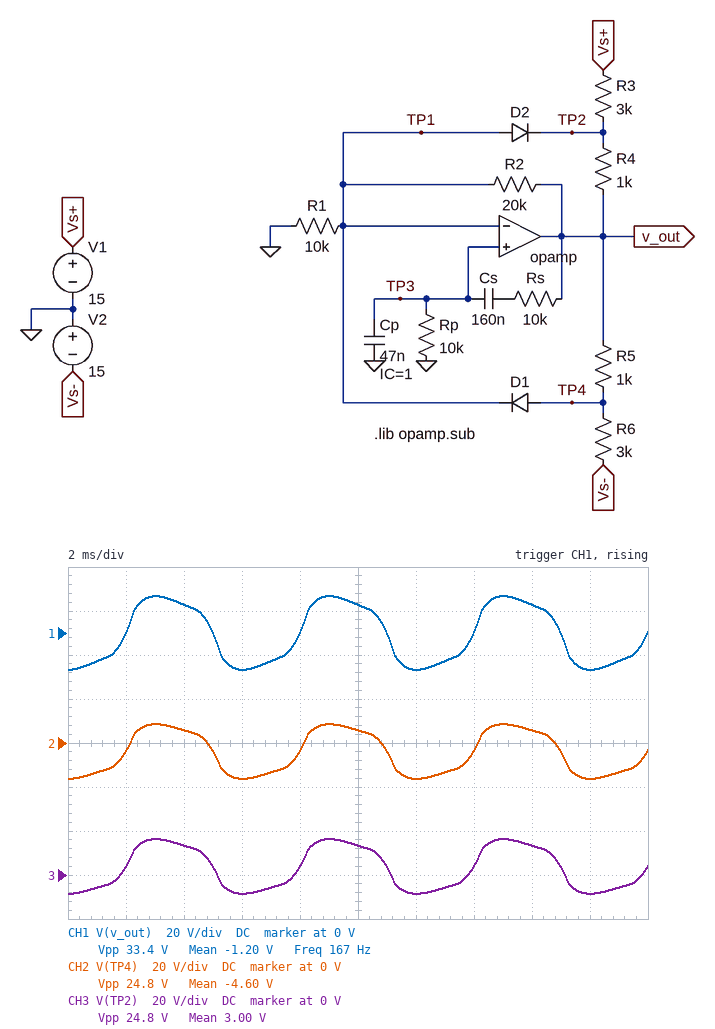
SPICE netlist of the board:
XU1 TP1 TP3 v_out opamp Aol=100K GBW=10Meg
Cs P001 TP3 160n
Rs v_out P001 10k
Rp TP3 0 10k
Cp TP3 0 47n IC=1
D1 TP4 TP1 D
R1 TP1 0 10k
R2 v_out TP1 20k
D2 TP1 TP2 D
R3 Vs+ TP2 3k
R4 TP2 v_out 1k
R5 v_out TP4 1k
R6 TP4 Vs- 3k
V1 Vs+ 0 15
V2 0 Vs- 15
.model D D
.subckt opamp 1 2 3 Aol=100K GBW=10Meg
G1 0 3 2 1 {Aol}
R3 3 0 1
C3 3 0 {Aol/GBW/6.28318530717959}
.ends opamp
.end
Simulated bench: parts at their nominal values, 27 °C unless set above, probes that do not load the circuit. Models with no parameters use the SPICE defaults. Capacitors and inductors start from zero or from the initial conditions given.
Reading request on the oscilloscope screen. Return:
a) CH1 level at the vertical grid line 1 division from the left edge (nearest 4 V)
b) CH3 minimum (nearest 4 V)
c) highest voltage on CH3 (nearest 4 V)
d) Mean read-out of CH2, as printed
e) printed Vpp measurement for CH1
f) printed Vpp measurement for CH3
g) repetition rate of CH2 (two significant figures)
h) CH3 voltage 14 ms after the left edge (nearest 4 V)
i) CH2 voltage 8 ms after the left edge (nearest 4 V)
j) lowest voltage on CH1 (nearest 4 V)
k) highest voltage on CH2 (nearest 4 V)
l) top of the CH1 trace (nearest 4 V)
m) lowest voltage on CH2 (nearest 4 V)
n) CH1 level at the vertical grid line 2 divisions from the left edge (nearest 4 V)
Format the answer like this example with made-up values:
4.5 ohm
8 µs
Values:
0 V
-8 V
16 V
-4.60 V
33.4 V
24.8 V
170 Hz
4 V
-4 V
-16 V
8 V
16 V
-16 V
12 V
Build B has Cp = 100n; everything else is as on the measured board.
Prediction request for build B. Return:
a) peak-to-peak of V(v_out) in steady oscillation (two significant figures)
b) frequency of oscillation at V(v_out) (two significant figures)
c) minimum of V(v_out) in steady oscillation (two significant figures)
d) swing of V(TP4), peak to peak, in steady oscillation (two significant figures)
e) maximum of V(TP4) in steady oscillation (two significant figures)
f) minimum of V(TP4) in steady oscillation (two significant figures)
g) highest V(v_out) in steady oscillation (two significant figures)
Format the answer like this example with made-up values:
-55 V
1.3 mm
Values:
26 V
120 Hz
-13 V
20 V
6.0 V
-14 V
13 V
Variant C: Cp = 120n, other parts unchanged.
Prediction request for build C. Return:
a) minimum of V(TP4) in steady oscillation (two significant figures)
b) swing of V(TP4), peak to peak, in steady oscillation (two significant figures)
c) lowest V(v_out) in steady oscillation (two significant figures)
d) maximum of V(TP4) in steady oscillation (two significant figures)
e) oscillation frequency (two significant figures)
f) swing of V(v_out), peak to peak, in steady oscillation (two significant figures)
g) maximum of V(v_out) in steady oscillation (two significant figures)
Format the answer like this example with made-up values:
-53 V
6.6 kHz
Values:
-13 V
18 V
-12 V
5.3 V
110 Hz
24 V
12 V
